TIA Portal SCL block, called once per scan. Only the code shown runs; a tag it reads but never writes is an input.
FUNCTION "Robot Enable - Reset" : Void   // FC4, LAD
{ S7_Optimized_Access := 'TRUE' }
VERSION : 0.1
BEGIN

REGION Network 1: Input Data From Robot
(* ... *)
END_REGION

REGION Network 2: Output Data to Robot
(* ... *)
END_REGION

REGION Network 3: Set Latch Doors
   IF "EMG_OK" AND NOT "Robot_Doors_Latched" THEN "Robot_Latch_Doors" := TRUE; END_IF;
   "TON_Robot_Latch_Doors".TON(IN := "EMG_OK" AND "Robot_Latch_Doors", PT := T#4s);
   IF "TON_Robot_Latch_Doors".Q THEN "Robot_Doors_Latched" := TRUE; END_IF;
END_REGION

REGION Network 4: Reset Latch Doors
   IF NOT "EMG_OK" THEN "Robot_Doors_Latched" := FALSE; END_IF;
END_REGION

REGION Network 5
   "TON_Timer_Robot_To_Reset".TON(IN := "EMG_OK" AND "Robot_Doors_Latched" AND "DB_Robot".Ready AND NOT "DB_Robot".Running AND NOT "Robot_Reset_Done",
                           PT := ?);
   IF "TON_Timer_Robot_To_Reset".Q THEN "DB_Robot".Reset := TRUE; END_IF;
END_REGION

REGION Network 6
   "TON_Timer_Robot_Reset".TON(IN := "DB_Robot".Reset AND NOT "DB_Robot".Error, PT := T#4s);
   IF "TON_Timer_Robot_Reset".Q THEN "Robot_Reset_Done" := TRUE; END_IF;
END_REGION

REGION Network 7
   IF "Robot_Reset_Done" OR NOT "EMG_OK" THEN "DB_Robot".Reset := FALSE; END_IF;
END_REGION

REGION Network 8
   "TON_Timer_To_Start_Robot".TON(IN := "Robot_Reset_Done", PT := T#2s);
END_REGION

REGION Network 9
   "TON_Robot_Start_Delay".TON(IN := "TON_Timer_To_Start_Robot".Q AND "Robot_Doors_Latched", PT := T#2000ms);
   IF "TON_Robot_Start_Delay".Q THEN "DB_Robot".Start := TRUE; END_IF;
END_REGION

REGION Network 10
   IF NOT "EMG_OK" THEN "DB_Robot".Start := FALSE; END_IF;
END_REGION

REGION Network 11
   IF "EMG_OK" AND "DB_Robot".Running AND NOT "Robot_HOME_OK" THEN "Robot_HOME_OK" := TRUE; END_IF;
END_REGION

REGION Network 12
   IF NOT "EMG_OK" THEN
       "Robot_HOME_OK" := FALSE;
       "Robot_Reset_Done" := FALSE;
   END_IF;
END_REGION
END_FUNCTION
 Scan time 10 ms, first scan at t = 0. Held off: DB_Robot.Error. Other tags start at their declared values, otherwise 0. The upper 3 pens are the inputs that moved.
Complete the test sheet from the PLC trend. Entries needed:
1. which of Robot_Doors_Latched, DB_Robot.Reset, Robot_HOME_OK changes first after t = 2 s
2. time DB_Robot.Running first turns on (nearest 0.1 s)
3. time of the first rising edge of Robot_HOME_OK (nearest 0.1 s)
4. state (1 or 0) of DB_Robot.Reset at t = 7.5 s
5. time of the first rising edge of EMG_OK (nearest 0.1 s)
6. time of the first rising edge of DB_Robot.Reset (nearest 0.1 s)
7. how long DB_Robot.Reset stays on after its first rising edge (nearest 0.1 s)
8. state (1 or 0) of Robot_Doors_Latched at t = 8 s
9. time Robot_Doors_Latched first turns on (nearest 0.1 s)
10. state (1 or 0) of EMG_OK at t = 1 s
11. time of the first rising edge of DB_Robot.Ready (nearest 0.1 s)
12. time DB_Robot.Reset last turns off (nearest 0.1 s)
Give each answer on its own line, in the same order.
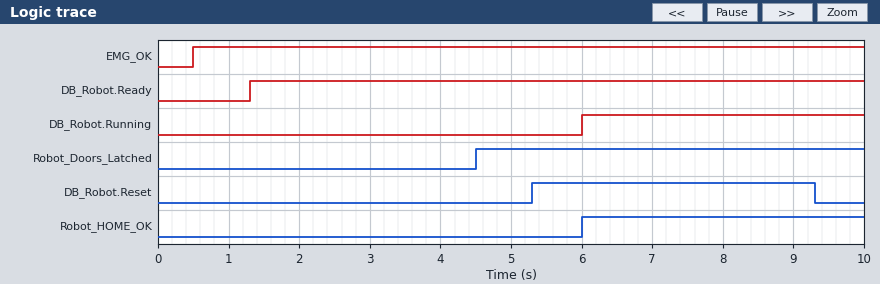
Robot_Doors_Latched
6.0 s
6.0 s
1
0.5 s
5.3 s
4.0 s
1
4.5 s
1
1.3 s
9.3 s
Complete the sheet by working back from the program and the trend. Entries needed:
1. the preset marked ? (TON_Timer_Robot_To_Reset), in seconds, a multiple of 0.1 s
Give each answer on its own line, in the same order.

0.8 s
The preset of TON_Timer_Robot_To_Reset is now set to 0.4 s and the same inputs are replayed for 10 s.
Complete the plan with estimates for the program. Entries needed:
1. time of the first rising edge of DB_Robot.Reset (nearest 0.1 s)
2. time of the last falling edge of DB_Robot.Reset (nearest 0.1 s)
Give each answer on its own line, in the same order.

4.9 s
8.9 s
